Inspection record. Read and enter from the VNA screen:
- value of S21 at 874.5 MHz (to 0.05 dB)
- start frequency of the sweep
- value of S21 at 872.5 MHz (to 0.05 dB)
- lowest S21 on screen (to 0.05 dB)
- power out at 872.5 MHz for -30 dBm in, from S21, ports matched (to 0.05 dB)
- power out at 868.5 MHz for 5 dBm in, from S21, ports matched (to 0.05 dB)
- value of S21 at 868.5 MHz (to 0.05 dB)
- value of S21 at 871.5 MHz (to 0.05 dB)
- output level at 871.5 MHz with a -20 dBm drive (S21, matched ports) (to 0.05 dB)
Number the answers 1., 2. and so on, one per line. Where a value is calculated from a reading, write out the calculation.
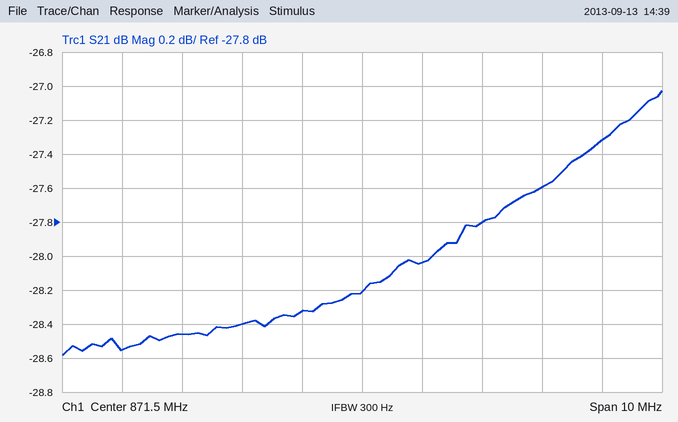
1. -27.60 dB
2. 866.5 MHz
3. -28.05 dB
4. -28.60 dB
5. -30 dBm + (-28.05 dB) = -58.05 dBm
6. 5 dBm + (-28.45 dB) = -23.45 dBm
7. -28.45 dB
8. -28.20 dB
9. -20 dBm + (-28.20 dB) = -48.20 dBm
